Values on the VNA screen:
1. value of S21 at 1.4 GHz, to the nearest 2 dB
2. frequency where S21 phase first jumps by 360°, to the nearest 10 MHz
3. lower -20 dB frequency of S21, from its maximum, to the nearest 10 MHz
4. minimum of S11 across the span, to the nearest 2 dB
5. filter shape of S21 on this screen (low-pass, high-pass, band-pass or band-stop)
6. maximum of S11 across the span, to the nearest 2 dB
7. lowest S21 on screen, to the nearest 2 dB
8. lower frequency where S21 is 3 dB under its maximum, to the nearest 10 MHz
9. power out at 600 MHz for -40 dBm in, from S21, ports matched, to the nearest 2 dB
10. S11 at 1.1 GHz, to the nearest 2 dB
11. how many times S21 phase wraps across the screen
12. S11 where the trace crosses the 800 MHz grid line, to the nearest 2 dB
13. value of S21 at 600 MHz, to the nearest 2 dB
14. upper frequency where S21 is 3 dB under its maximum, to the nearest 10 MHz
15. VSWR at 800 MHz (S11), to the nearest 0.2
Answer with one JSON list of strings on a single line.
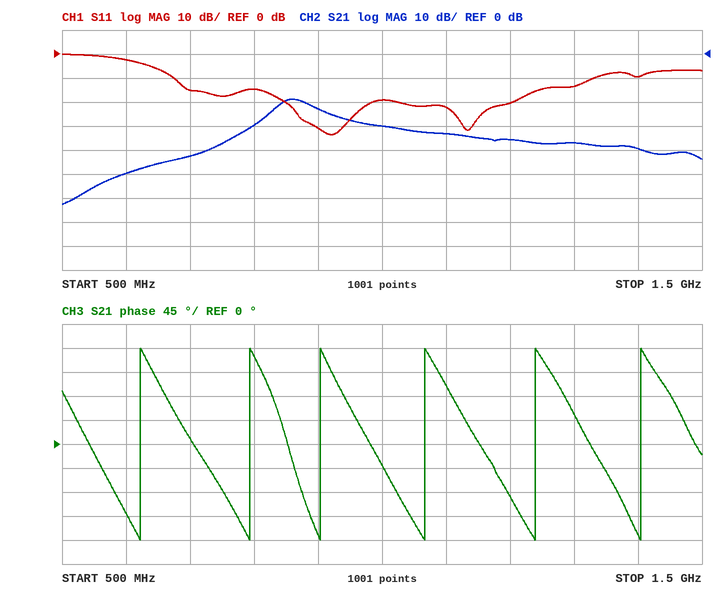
["-40 dB", "620 MHz", "740 MHz", "-34 dB", "band-pass", "0 dB", "-62 dB", "840 MHz", "-90 dBm", "-22 dB", "6", "-14 dB", "-50 dB", "890 MHz", "1.4"]
